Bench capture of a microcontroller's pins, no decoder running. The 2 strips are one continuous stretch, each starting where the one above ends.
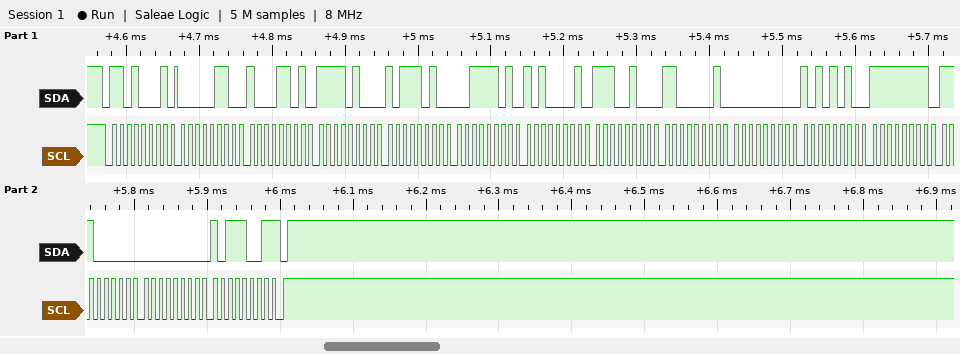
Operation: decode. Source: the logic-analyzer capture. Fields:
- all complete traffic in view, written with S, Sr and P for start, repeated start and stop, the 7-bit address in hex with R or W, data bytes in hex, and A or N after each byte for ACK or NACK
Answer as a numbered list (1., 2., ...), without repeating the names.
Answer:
1. S 68R A 06 A 8D A F4 A BA A 3D A A1 A E4 A C1 A 00 A AA A FF A E0 A 00 A B9 N P
